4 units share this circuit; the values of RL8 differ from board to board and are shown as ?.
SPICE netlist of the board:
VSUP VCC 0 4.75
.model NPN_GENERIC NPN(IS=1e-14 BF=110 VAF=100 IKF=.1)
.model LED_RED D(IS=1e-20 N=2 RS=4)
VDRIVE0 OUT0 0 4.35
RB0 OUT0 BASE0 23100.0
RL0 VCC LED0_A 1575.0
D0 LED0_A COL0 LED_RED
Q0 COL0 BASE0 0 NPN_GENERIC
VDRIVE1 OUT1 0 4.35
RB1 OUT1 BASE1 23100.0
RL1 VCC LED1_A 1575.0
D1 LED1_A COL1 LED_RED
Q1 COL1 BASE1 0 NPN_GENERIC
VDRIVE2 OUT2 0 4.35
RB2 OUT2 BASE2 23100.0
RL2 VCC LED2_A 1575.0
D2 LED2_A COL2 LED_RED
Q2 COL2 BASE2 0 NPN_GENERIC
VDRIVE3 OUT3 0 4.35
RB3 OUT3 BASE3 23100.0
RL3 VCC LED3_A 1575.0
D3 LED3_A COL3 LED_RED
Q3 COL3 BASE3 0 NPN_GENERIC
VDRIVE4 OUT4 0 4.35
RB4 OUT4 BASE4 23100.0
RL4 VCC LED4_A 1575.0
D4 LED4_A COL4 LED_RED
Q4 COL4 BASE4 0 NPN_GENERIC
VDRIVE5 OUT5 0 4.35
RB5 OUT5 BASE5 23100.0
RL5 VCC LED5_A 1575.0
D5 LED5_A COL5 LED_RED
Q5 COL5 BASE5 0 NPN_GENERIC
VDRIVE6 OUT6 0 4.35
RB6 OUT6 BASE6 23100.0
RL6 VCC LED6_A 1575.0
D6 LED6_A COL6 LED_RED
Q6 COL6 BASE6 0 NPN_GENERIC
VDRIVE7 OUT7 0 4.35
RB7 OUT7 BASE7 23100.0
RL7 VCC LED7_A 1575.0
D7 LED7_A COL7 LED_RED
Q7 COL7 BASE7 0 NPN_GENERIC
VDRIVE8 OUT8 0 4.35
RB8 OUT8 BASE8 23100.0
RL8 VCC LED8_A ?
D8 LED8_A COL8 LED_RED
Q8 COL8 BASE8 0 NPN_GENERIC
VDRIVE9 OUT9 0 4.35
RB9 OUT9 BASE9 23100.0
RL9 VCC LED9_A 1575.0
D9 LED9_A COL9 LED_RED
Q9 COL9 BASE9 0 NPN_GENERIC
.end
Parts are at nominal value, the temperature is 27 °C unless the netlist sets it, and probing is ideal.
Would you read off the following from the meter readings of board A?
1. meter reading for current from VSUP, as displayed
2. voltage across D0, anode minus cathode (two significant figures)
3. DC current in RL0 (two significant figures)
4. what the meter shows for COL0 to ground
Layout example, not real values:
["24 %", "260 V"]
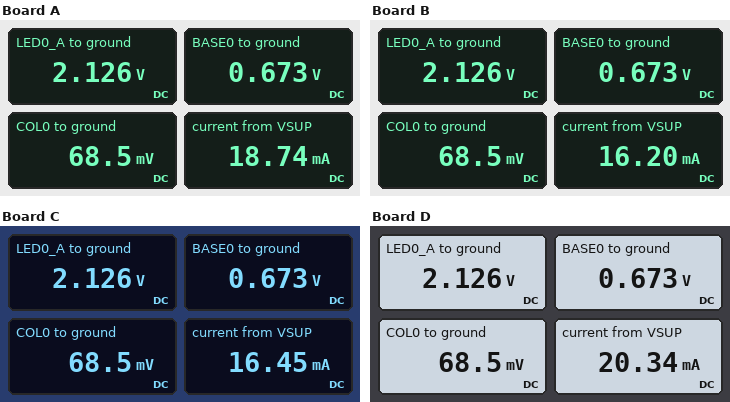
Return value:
["18.74 mA", "2.1 V", "1.7 mA", "68.5 mV"]
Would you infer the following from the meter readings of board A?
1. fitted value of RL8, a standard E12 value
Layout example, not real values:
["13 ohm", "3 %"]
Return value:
["680 Ω"]
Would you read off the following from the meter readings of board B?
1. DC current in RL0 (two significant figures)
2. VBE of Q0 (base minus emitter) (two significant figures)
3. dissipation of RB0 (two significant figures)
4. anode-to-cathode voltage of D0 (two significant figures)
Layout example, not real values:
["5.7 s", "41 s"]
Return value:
["1.7 mA", "670 mV", "590 µW", "2.1 V"]
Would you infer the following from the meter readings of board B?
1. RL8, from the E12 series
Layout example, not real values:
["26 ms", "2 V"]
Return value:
["2.2 kΩ"]
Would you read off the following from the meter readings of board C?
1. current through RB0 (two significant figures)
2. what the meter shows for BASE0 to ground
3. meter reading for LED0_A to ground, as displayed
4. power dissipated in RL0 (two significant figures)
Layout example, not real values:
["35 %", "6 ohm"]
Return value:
["160 µA", "0.673 V", "2.126 V", "4.4 mW"]
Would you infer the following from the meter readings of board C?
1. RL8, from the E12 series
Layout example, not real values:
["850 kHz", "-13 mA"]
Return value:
["1.8 kΩ"]
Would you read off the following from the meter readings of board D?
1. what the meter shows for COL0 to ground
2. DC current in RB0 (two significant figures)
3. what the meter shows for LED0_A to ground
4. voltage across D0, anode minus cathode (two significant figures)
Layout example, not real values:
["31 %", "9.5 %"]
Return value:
["68.5 mV", "160 µA", "2.126 V", "2.1 V"]
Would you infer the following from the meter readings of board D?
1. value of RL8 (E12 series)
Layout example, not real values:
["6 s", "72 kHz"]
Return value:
["470 Ω"]
